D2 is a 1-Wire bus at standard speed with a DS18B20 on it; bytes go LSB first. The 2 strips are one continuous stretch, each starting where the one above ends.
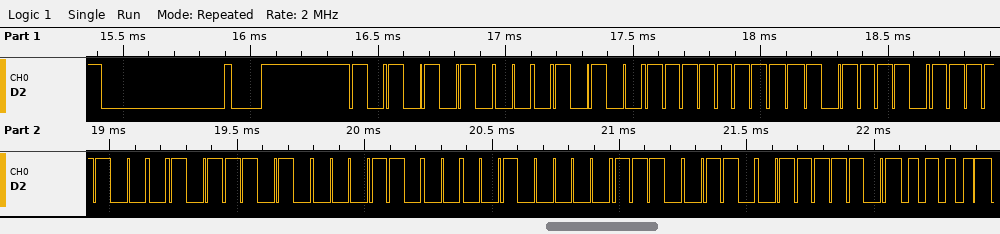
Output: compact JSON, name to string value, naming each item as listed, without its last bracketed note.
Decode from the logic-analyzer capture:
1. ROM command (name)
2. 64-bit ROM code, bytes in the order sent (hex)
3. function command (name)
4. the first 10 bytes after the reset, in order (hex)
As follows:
{"ROM command": "Match ROM", "64-bit ROM code, bytes in the order sent": "28 FF 7B 1F 5D 18 04 67", "function command": "Read Scratchpad", "the first 10 bytes after the reset, in order": "55 28 FF 7B 1F 5D 18 04 67 BE"}
